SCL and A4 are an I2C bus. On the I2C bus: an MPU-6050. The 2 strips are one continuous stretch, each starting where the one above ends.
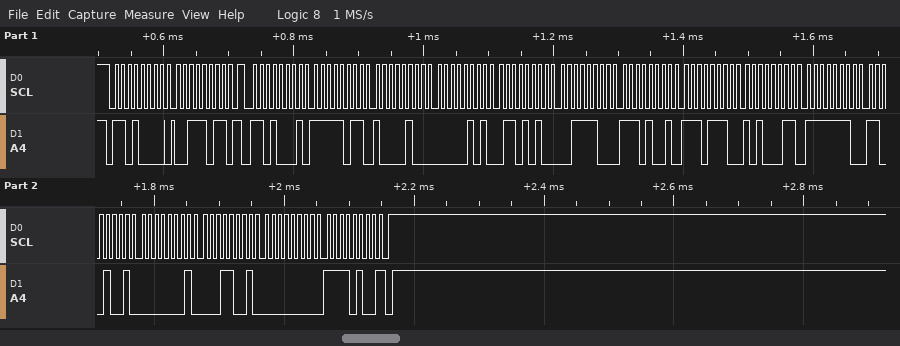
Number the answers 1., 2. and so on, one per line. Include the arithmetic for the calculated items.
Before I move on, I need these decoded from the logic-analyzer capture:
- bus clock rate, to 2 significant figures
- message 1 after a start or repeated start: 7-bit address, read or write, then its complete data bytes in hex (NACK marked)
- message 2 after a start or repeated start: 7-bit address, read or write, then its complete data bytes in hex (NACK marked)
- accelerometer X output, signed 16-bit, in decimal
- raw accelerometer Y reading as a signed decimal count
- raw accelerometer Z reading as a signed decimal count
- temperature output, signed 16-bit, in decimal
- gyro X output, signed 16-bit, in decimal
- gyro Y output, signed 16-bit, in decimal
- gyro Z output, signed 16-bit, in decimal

1. 100 kHz
2. 0x68 write: 3B
3. 0x68 read: FB 84 05 6A 3C E9 EE A3 FE C9 01 19 00 F4 NACK
4. 0xFB84 = -1148
5. 0x056A = 1386
6. 0x3CE9 = 15593
7. 0xEEA3 = -4445
8. 0xFEC9 = -311
9. 0x0119 = 281
10. 0x00F4 = 244
